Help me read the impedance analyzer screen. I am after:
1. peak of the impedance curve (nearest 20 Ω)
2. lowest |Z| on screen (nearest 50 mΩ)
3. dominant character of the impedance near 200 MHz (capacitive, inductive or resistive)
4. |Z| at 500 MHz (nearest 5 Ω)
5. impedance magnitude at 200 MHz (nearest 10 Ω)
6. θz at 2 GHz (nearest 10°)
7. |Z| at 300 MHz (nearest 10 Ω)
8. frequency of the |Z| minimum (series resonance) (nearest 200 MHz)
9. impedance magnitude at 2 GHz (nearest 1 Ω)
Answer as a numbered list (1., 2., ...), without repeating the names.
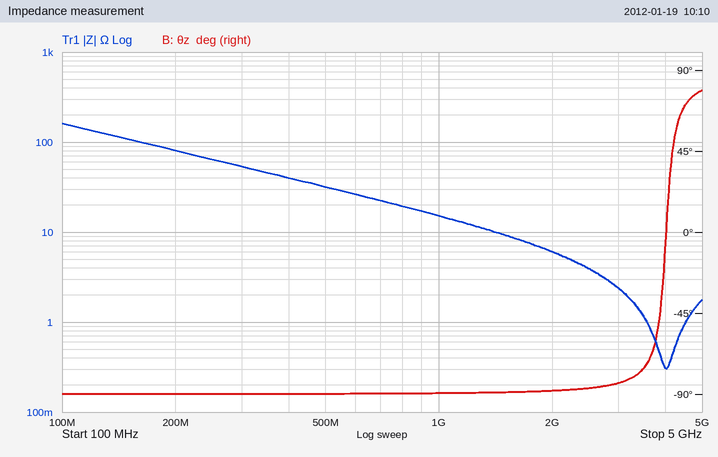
1. 160 Ω
2. 300 mΩ
3. capacitive
4. 30 Ω
5. 80 Ω
6. -90°
7. 50 Ω
8. 4.0 GHz
9. 6 Ω
